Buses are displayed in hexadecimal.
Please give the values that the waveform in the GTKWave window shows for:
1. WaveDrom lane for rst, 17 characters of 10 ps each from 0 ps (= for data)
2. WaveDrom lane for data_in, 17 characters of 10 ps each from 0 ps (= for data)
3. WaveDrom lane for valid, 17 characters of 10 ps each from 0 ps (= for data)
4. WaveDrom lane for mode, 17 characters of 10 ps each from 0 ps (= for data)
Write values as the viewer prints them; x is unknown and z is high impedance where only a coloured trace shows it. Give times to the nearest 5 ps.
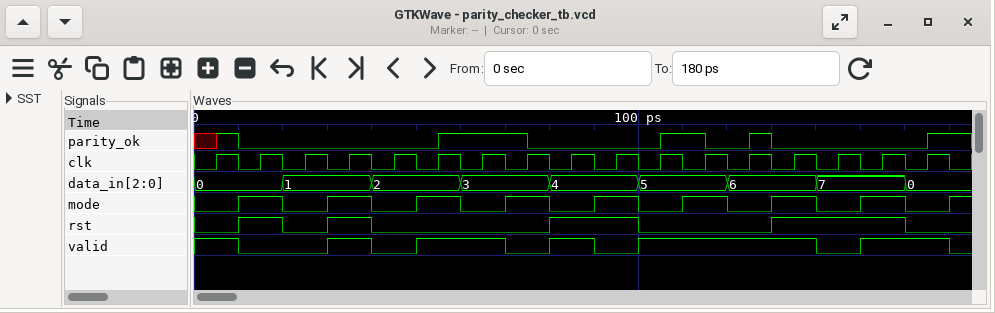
{name: 'rst', wave: '01010...1.0..1..0'}
{name: 'data_in', wave: '=.=.=.=.=.=.=.=.=', data: '0 1 2 3 4 5 6 7 0'}
{name: 'valid', wave: '10.101.0101...01.'}
{name: 'mode', wave: '01010101010101010'}
